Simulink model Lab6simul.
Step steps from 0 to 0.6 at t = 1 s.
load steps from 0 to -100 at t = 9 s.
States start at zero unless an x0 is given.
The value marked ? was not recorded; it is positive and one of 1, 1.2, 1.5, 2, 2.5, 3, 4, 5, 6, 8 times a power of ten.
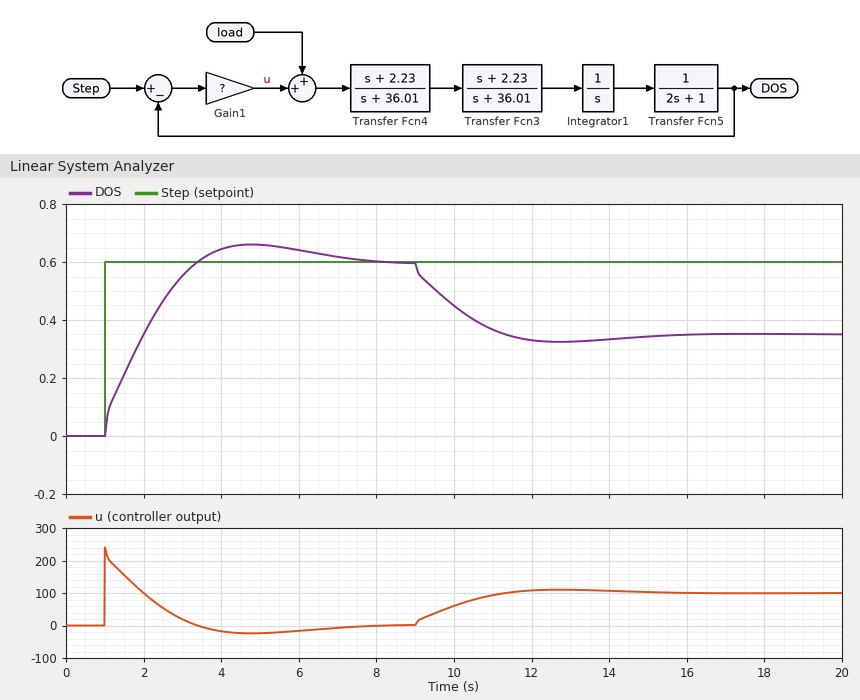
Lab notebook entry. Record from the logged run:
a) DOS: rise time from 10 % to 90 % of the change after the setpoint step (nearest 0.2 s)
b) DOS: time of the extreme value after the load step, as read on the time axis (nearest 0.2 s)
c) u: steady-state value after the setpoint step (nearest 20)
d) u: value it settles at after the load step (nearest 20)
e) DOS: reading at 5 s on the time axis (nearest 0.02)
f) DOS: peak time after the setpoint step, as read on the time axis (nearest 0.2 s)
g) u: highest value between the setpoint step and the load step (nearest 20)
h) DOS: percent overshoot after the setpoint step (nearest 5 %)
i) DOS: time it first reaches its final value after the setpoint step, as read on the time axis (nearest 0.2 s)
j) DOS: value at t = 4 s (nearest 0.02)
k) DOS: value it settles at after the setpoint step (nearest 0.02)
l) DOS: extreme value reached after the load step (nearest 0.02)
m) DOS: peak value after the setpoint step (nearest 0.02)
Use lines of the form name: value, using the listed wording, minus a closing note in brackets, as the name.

DOS: rise time from 10 % to 90 % of the change after the setpoint step: 1.8 s
DOS: time of the extreme value after the load step, as read on the time axis: 12.8 s
u: steady-state value after the setpoint step: 0
u: value it settles at after the load step: 100
DOS: reading at 5 s on the time axis: 0.66
DOS: peak time after the setpoint step, as read on the time axis: 4.8 s
u: highest value between the setpoint step and the load step: 240
DOS: percent overshoot after the setpoint step: 10 %
DOS: time it first reaches its final value after the setpoint step, as read on the time axis: 3.4 s
DOS: value at t = 4 s: 0.64
DOS: value it settles at after the setpoint step: 0.60
DOS: extreme value reached after the load step: 0.32
DOS: peak value after the setpoint step: 0.66
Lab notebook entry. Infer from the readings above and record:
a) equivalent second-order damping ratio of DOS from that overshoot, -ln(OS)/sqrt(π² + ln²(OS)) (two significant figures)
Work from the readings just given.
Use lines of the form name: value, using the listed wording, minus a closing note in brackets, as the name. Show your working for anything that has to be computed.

equivalent second-order damping ratio of DOS from that overshoot, -ln(OS)/sqrt(π² + ln²(OS)): ln(0.1) = -2.303; 2.303 / sqrt(9.870 + 5.302) = 0.59
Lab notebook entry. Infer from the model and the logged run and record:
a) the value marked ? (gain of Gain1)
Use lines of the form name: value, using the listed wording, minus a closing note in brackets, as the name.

the value marked ?: 400
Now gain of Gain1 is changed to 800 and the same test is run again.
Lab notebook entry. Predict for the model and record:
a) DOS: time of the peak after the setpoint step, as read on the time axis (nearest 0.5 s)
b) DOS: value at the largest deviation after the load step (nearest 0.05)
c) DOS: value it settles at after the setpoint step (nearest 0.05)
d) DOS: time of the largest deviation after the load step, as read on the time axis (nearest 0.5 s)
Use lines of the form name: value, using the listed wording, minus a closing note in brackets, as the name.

DOS: time of the peak after the setpoint step, as read on the time axis: 3.5 s
DOS: value at the largest deviation after the load step: 0.45
DOS: value it settles at after the setpoint step: 0.60
DOS: time of the largest deviation after the load step, as read on the time axis: 11.5 s
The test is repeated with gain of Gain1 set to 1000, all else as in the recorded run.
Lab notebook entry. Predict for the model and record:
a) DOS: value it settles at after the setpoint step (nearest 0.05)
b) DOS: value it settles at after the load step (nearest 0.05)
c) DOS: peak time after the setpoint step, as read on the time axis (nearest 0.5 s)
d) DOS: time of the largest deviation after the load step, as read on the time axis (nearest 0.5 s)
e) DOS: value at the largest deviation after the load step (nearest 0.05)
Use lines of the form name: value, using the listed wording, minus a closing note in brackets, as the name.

DOS: value it settles at after the setpoint step: 0.60
DOS: value it settles at after the load step: 0.50
DOS: peak time after the setpoint step, as read on the time axis: 3.5 s
DOS: time of the largest deviation after the load step, as read on the time axis: 11.5 s
DOS: value at the largest deviation after the load step: 0.50
